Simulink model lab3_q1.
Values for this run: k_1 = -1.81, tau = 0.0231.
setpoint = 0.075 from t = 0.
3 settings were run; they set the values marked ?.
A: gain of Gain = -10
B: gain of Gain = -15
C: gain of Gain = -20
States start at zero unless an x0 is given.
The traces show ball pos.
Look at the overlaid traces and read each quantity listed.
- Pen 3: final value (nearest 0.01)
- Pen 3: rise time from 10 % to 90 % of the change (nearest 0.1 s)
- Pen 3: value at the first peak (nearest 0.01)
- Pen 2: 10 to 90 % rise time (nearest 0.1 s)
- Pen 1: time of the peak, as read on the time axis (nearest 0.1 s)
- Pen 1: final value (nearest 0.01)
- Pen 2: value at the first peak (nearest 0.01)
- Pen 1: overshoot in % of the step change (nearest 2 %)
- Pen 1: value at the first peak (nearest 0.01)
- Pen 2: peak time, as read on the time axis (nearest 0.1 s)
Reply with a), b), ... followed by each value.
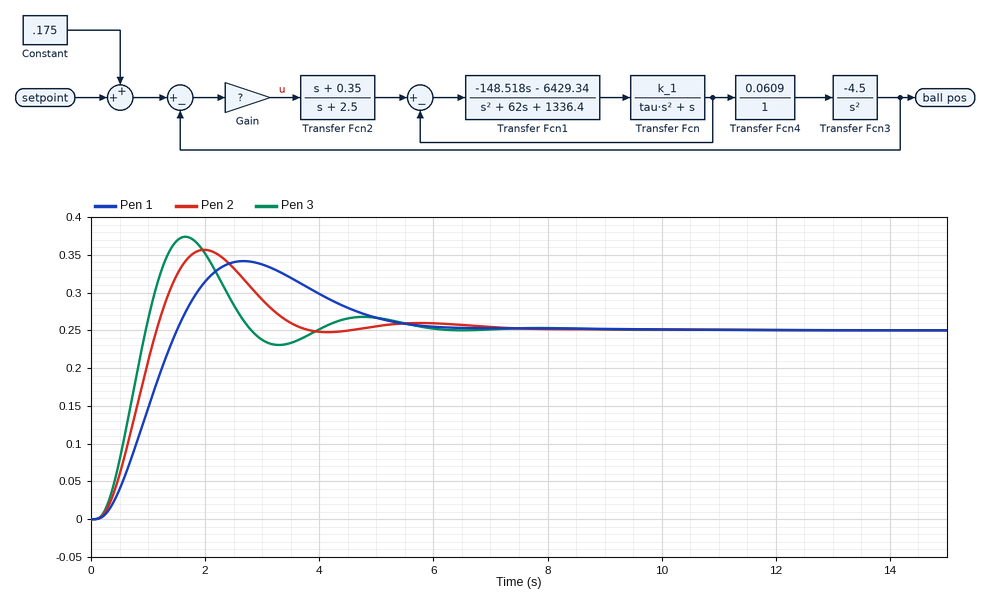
a) 0.25
b) 0.6 s
c) 0.37
d) 0.7 s
e) 2.7 s
f) 0.25
g) 0.36
h) 36 %
i) 0.34
j) 2.0 s
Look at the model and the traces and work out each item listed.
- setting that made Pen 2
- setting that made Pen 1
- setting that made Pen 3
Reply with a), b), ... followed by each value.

a) B
b) A
c) C
